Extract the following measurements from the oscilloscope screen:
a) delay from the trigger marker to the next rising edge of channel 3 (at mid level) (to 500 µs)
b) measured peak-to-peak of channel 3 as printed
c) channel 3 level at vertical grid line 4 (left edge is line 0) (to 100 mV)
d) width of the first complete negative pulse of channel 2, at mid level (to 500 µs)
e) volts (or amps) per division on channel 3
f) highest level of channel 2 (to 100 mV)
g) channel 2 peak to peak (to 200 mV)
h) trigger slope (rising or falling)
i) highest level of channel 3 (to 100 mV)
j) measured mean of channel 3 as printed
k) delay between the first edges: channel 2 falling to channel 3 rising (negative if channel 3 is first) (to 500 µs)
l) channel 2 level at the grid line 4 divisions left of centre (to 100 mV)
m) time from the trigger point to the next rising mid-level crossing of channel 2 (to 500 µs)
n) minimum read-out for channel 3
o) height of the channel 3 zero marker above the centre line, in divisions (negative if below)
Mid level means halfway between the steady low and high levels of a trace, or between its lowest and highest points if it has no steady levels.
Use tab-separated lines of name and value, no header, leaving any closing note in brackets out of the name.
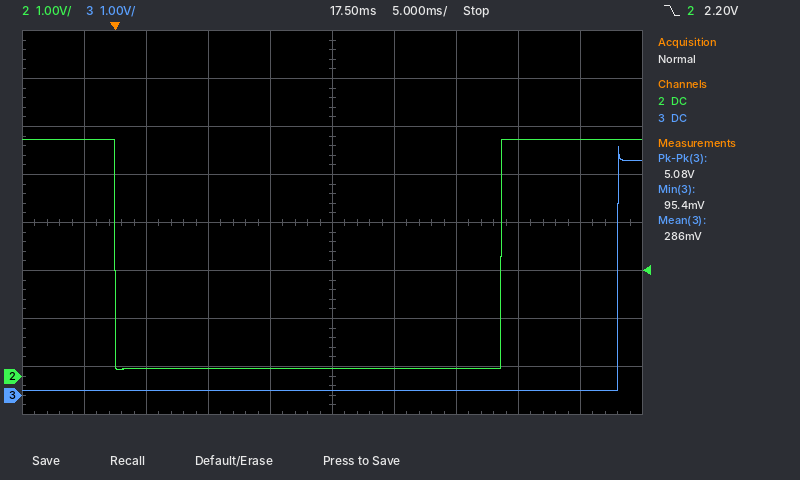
delay from the trigger marker to the next rising edge of channel 3 (at mid level)	40.5 ms
measured peak-to-peak of channel 3 as printed	5.08 V
channel 3 level at vertical grid line 4 (left edge is line 0)	100 mV
width of the first complete negative pulse of channel 2, at mid level	31.0 ms
volts (or amps) per division on channel 3	1 V
highest level of channel 2	4.9 V
channel 2 peak to peak	4.8 V
trigger slope	falling
highest level of channel 3	5.2 V
measured mean of channel 3 as printed	286 mV
delay between the first edges: channel 2 falling to channel 3 rising (negative if channel 3 is first)	+40.5 ms
channel 2 level at the grid line 4 divisions left of centre	4.9 V
time from the trigger point to the next rising mid-level crossing of channel 2	31.0 ms
minimum read-out for channel 3	95.4 mV
height of the channel 3 zero marker above the centre line, in divisions	-3.6 div
